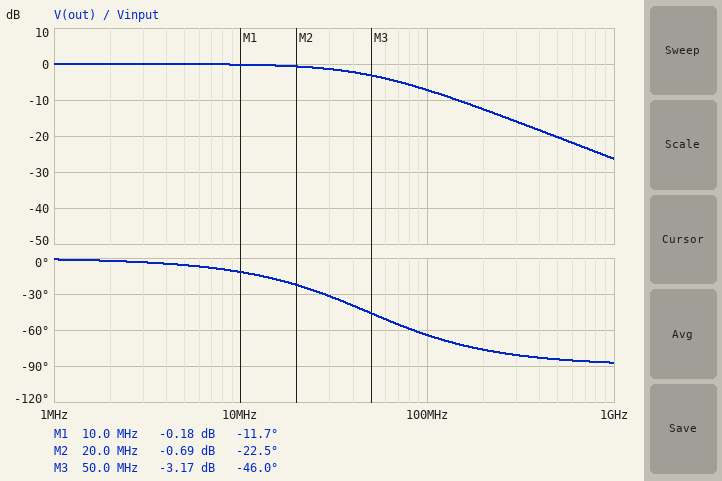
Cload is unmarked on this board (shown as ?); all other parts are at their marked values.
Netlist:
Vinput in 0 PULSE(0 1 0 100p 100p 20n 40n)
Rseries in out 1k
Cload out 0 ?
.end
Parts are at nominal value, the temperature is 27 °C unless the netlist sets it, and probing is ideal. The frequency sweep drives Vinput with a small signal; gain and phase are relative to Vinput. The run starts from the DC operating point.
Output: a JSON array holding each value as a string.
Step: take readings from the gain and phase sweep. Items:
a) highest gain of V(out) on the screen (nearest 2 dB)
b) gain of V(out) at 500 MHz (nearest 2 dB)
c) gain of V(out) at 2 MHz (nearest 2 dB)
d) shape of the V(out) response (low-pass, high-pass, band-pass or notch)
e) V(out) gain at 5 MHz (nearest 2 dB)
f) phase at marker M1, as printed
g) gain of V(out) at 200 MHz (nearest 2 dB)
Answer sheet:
["0 dB", "-20 dB", "0 dB", "low-pass", "0 dB", "-11.7 deg", "-12 dB"]
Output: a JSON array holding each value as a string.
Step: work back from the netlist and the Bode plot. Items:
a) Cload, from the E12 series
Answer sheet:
["3.3 pF"]
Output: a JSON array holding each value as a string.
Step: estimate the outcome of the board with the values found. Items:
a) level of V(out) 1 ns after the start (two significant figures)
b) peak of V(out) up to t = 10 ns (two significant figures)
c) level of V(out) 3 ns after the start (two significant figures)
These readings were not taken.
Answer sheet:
["250 mV", "950 mV", "590 mV"]
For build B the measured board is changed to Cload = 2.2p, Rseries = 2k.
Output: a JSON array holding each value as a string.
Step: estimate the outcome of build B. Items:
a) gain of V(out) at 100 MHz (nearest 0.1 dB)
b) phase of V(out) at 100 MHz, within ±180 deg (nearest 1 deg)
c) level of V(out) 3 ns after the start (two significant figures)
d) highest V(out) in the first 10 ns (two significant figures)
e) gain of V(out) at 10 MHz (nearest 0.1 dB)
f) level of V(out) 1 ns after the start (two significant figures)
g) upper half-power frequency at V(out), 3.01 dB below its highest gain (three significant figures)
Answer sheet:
["-9.4 dB", "-70 deg", "490 mV", "900 mV", "-0.3 dB", "190 mV", "36.2 MHz"]
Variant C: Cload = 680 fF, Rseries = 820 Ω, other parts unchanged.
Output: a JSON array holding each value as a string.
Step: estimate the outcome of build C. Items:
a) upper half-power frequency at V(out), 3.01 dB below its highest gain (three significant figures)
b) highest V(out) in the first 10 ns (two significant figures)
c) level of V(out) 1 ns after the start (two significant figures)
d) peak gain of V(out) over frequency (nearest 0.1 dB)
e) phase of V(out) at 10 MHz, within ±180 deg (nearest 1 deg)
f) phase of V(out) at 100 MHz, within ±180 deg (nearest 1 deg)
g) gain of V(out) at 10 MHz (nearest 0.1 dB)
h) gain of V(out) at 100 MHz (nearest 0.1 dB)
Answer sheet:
["285 MHz", "1.0 V", "820 mV", "0 dB", "-2 deg", "-19 deg", "0 dB", "-0.5 dB"]
